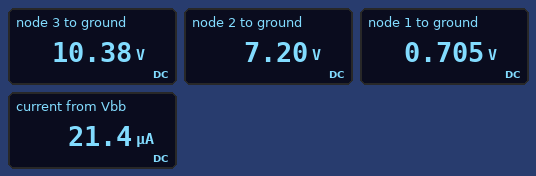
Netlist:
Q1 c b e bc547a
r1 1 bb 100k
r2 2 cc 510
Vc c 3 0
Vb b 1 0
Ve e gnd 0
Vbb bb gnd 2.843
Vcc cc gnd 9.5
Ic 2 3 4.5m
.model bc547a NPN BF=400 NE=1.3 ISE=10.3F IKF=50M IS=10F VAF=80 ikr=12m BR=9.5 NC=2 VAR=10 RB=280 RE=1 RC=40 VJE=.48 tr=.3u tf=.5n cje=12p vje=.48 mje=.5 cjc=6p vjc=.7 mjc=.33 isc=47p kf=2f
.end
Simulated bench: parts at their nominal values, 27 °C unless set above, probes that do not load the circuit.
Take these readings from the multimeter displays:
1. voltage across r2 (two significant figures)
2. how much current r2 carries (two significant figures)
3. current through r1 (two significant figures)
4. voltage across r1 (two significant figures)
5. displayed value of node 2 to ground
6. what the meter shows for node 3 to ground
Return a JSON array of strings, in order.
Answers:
["2.3 V", "4.5 mA", "21 µA", "2.1 V", "7.20 V", "10.38 V"]
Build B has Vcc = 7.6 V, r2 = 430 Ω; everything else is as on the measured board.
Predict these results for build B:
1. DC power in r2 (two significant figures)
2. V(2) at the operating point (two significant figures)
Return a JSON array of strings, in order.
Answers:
["8.7 mW", "5.7 V"]
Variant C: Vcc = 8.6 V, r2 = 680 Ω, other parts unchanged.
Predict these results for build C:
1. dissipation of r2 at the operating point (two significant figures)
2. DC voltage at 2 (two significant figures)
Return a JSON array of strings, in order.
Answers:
["14 mW", "5.5 V"]
